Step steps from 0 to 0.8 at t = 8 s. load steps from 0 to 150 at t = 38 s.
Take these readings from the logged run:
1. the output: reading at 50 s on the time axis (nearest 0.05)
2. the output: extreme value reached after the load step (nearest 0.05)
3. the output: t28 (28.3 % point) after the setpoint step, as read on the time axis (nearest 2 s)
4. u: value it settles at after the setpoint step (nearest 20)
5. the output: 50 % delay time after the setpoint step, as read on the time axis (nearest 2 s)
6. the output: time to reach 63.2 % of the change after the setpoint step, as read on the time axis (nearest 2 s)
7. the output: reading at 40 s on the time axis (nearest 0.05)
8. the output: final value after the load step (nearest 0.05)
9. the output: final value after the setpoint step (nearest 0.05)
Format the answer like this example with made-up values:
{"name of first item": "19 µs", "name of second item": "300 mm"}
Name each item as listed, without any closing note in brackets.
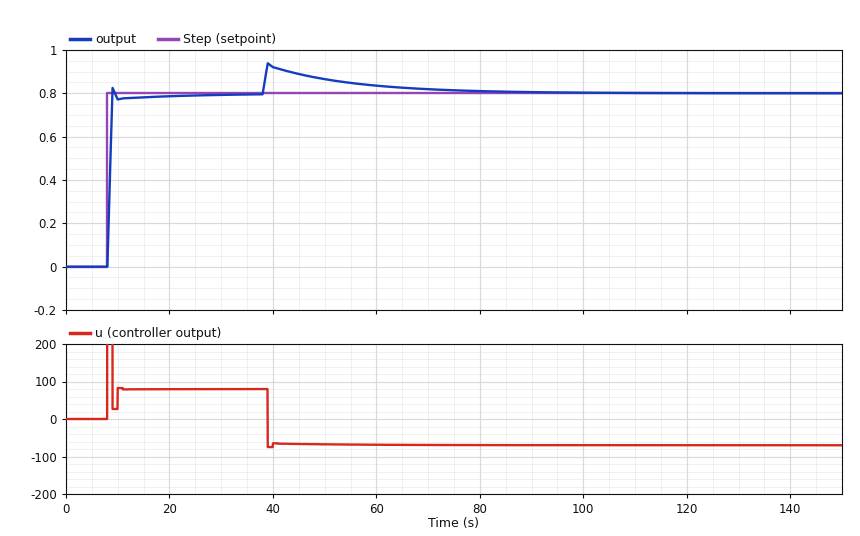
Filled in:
{"the output: reading at 50 s on the time axis": "0.85", "the output: extreme value reached after the load step": "0.95", "the output: t28 (28.3 % point) after the setpoint step, as read on the time axis": "8 s", "u: value it settles at after the setpoint step": "80", "the output: 50 % delay time after the setpoint step, as read on the time axis": "8 s", "the output: time to reach 63.2 % of the change after the setpoint step, as read on the time axis": "8 s", "the output: reading at 40 s on the time axis": "0.90", "the output: final value after the load step": "0.80", "the output: final value after the setpoint step": "0.80"}
